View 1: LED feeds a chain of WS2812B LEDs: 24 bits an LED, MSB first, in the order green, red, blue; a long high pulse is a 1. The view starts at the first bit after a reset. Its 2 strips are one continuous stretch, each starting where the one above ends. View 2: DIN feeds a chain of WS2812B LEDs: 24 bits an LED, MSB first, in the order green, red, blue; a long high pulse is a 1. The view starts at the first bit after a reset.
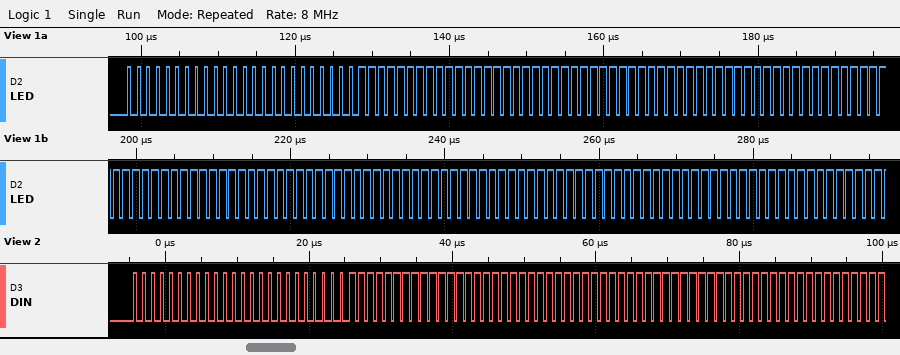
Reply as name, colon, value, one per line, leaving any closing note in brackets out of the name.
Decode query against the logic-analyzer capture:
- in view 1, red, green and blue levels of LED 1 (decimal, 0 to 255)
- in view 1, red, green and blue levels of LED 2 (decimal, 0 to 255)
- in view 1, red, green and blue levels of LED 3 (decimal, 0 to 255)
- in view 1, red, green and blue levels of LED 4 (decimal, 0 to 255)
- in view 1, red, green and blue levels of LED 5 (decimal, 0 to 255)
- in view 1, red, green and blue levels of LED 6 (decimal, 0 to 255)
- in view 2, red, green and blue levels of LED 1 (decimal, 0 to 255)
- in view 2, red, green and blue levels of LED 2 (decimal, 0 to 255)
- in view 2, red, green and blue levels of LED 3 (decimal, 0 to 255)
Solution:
in view 1, red, green and blue levels of LED 1: 0, 0, 0
in view 1, red, green and blue levels of LED 2: 255, 255, 255
in view 1, red, green and blue levels of LED 3: 255, 255, 255
in view 1, red, green and blue levels of LED 4: 255, 255, 255
in view 1, red, green and blue levels of LED 5: 255, 255, 255
in view 1, red, green and blue levels of LED 6: 255, 255, 255
in view 2, red, green and blue levels of LED 1: 0, 0, 0
in view 2, red, green and blue levels of LED 2: 255, 255, 255
in view 2, red, green and blue levels of LED 3: 255, 255, 255
